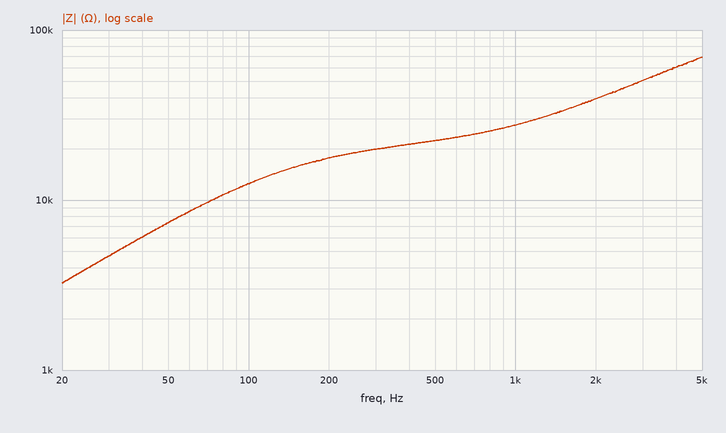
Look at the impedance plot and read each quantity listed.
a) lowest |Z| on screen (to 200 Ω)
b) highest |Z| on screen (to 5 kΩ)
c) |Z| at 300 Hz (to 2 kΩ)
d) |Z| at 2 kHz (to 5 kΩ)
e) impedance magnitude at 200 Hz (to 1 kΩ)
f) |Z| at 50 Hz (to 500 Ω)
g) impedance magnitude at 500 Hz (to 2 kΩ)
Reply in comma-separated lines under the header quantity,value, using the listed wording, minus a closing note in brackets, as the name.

quantity,value
lowest |Z| on screen,3.2 kΩ
highest |Z| on screen,70 kΩ
|Z| at 300 Hz,20 kΩ
|Z| at 2 kHz,40 kΩ
impedance magnitude at 200 Hz,18 kΩ
|Z| at 50 Hz,7.5 kΩ
impedance magnitude at 500 Hz,22 kΩ
